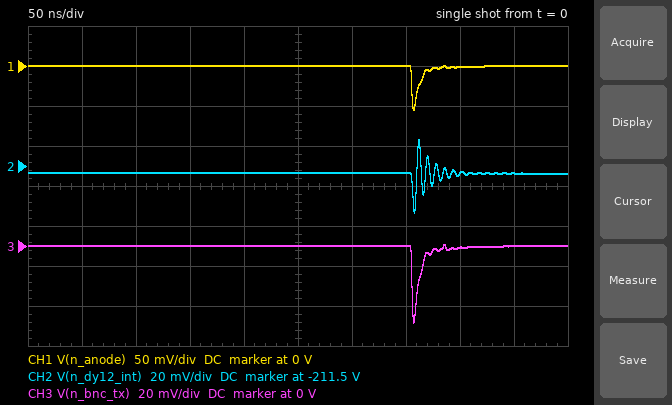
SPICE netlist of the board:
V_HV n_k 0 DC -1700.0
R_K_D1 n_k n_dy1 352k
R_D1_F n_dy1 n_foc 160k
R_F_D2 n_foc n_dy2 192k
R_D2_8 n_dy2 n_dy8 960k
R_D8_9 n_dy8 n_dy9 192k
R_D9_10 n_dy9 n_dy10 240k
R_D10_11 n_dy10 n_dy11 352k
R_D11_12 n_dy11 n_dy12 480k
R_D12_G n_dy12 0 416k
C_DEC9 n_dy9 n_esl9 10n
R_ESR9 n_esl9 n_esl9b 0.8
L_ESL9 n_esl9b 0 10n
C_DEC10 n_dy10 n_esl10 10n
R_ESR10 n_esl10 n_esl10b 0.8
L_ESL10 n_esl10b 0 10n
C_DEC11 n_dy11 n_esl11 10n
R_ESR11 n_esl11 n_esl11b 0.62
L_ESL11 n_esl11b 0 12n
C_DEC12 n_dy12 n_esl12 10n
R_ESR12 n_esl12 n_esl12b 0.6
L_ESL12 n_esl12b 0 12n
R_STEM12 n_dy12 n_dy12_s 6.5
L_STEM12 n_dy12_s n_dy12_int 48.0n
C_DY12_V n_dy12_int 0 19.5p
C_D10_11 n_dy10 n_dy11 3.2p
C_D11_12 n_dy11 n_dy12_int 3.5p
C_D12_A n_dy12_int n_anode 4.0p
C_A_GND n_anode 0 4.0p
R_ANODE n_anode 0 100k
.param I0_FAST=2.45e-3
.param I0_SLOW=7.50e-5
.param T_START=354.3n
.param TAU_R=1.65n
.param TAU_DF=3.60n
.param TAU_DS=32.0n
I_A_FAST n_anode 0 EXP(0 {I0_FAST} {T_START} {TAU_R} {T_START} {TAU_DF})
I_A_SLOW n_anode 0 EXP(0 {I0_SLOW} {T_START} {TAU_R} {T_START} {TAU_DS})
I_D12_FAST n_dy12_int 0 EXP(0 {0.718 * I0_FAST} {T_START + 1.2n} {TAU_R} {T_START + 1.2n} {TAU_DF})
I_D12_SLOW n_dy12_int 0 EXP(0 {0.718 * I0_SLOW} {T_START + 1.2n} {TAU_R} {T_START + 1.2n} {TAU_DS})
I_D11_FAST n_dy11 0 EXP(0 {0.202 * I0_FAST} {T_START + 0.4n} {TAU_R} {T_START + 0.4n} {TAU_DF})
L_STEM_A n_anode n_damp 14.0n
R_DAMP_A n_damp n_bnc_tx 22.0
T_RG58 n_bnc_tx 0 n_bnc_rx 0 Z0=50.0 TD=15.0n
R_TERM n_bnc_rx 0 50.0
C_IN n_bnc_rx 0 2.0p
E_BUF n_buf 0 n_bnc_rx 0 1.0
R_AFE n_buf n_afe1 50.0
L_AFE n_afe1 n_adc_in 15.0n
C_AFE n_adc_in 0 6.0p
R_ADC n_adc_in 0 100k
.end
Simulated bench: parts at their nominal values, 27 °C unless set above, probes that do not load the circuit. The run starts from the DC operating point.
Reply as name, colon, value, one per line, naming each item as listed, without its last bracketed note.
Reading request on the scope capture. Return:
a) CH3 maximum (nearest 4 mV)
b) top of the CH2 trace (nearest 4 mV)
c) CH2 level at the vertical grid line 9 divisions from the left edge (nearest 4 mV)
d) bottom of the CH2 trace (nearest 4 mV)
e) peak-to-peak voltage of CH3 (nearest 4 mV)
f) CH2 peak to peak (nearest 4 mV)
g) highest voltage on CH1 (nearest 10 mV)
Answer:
CH3 maximum: 0 V
top of the CH2 trace: -211.468 V
CH2 level at the vertical grid line 9 divisions from the left edge: -211.484 V
bottom of the CH2 trace: -211.504 V
peak-to-peak voltage of CH3: 40 mV
CH2 peak to peak: 36 mV
highest voltage on CH1: 0 V
